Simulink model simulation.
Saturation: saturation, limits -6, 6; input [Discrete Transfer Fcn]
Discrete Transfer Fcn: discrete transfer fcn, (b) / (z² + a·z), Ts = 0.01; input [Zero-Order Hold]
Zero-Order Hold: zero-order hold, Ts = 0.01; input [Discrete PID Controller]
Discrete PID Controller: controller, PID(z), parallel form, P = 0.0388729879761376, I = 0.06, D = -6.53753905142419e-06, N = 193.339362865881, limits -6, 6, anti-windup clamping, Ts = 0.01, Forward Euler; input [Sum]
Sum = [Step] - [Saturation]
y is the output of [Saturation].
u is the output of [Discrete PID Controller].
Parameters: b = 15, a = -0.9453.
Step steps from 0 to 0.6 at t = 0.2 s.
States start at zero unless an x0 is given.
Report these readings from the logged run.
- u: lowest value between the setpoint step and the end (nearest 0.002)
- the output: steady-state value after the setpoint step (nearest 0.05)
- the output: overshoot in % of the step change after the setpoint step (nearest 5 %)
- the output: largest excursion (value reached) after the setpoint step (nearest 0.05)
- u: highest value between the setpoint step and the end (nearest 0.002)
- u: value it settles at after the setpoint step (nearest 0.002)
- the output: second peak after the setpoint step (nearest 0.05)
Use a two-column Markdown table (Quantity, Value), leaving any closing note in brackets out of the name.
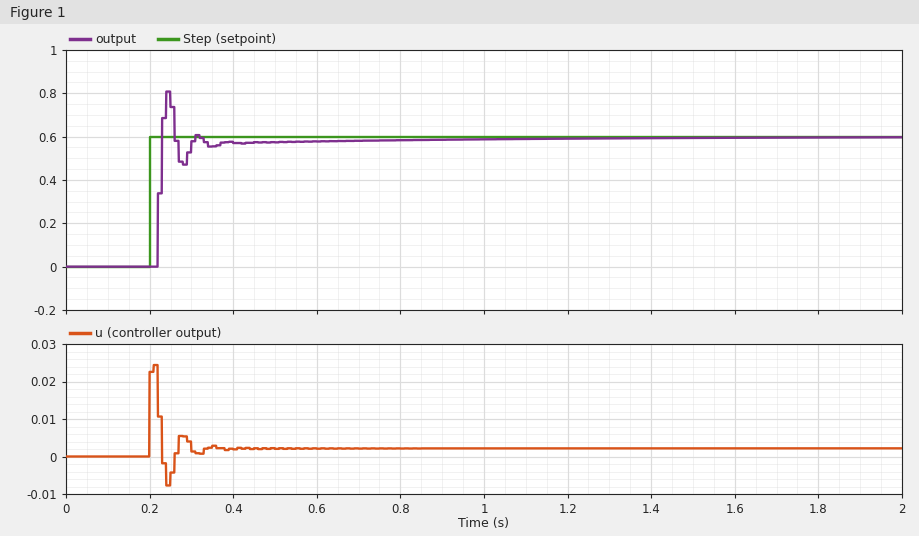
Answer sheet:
| Quantity | Value |
|---|---|
| u: lowest value between the setpoint step and the end | -0.008 |
| the output: steady-state value after the setpoint step | 0.60 |
| the output: overshoot in % of the step change after the setpoint step | 35 % |
| the output: largest excursion (value reached) after the setpoint step | 0.80 |
| u: highest value between the setpoint step and the end | 0.024 |
| u: value it settles at after the setpoint step | 0.002 |
| the output: second peak after the setpoint step | 0.60 |
